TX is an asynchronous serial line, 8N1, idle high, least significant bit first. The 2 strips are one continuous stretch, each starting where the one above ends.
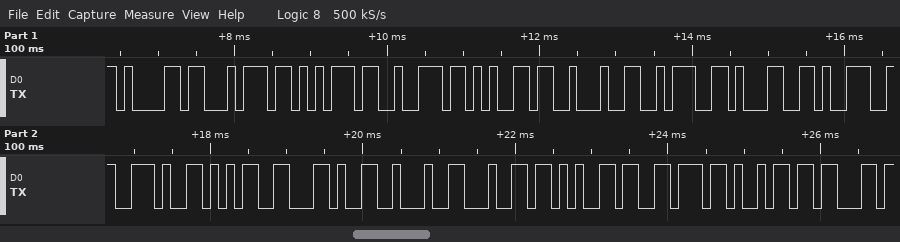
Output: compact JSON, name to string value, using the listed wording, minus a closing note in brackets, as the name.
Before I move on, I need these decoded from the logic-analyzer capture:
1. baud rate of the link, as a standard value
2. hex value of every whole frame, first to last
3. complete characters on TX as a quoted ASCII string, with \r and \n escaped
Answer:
{"baud rate of the link, as a standard value": "9600 baud", "hex value of every whole frame, first to last": "61 74 75 72 65 22 3A 31 39 2E 35 2C 22 64 65 76 69 63", "complete characters on TX as a quoted ASCII string, with \\r and \\n escaped": "\"ature\\\":19.5,\\\"devic\""}
